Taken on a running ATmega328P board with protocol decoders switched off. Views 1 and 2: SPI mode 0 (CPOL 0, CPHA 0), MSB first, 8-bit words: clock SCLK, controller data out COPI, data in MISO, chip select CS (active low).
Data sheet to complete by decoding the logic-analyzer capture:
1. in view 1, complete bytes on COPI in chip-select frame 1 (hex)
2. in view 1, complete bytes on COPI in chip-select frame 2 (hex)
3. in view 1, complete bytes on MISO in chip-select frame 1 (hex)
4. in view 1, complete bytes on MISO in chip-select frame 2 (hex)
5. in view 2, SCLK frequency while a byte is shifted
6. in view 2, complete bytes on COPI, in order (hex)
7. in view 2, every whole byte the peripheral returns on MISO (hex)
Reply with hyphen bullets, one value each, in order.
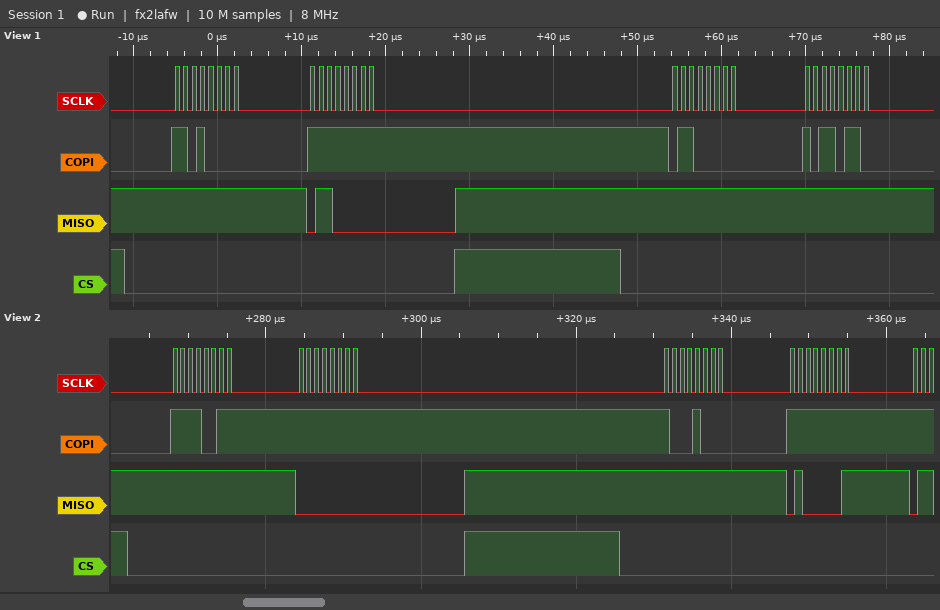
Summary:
- D0 FF
- 60 B6
- FF 60
- FF FF
- 1 MHz
- F3 FF 88 FF
- FF 00 FF 41
